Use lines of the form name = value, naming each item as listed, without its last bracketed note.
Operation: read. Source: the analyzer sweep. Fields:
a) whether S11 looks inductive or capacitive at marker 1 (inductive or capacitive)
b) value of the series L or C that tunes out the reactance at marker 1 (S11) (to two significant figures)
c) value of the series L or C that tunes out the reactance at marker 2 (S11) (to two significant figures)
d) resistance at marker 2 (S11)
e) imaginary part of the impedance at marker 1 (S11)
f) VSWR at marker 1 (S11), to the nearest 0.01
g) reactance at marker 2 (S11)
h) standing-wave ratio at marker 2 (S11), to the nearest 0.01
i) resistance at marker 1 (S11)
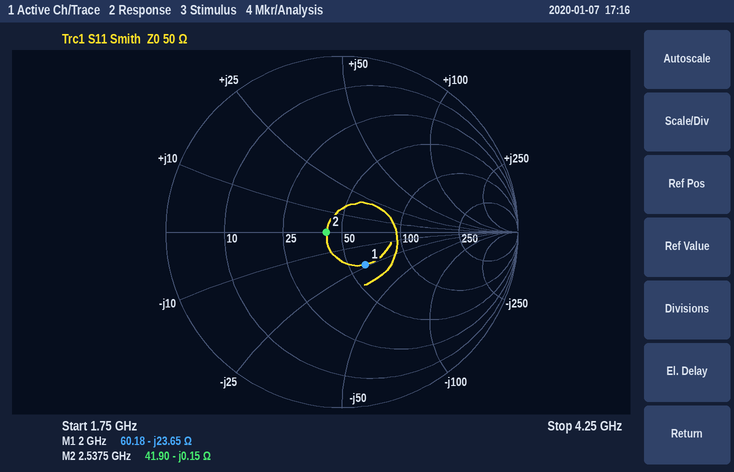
whether S11 looks inductive or capacitive at marker 1 = capacitive
value of the series L or C that tunes out the reactance at marker 1 (S11) = 1.9 nH
value of the series L or C that tunes out the reactance at marker 2 (S11) = 9.4 pH
resistance at marker 2 = 41.90 Ω
imaginary part of the impedance at marker 1 = -23.65 Ω
VSWR at marker 1 (S11), to the nearest 0.01 = 1.59
reactance at marker 2 = -0.15 Ω
standing-wave ratio at marker 2 (S11), to the nearest 0.01 = 1.19
resistance at marker 1 = 60.18 Ω
